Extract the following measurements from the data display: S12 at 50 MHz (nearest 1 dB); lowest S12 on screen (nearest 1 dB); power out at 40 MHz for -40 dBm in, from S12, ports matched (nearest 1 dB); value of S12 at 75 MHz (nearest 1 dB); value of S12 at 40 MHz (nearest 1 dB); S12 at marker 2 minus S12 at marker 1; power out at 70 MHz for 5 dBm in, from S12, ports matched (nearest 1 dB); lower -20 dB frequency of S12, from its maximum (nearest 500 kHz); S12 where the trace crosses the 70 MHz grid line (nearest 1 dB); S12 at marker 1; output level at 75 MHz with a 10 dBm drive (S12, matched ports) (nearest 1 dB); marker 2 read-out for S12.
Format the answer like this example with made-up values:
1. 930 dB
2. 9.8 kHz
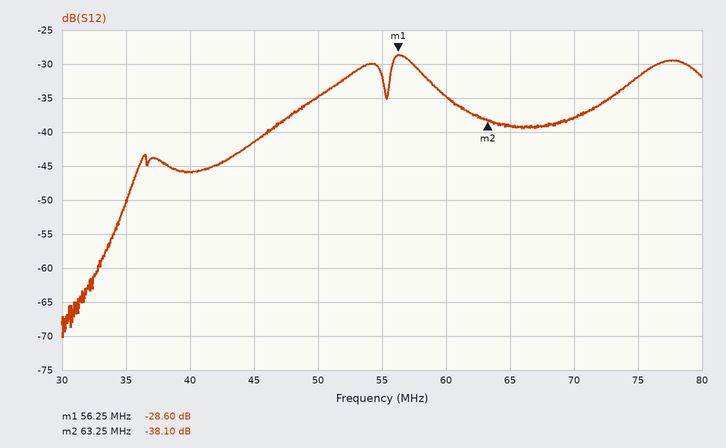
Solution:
1. -35 dB
2. -70 dB
3. -86 dBm
4. -32 dB
5. -46 dB
6. -9.50 dB
7. -33 dBm
8. 35.5 MHz
9. -38 dB
10. -28.60 dB
11. -22 dBm
12. -38.10 dB
